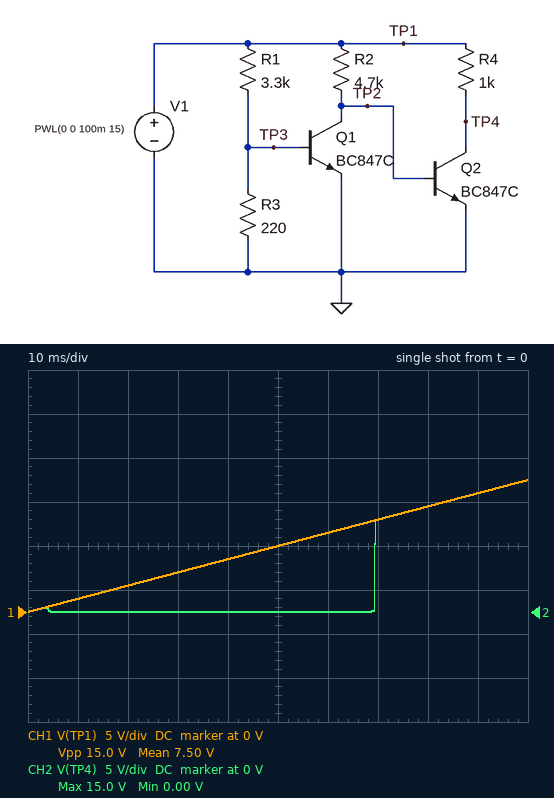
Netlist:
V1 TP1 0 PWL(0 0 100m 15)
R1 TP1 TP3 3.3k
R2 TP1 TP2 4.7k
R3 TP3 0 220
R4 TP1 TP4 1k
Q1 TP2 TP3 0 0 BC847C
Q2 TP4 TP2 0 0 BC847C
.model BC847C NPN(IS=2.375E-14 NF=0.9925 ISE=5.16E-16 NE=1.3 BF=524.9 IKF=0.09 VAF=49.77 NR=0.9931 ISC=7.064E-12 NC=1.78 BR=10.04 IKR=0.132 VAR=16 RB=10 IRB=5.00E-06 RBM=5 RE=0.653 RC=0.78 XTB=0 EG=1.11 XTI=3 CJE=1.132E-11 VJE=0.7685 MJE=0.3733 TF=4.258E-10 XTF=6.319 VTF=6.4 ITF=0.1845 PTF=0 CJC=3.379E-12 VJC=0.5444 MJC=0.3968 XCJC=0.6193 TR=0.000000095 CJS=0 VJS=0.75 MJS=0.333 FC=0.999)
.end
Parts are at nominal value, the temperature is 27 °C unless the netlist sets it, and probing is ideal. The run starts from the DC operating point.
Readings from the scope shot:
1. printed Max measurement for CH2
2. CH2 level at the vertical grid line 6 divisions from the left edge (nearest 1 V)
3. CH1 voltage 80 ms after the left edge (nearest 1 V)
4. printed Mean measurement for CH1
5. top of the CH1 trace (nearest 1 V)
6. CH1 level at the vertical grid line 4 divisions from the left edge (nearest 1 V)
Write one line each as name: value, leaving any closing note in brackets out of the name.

printed Max measurement for CH2: 15.0 V
CH2 level at the vertical grid line 6 divisions from the left edge: 0 V
CH1 voltage 80 ms after the left edge: 12 V
printed Mean measurement for CH1: 7.50 V
top of the CH1 trace: 15 V
CH1 level at the vertical grid line 4 divisions from the left edge: 6 V
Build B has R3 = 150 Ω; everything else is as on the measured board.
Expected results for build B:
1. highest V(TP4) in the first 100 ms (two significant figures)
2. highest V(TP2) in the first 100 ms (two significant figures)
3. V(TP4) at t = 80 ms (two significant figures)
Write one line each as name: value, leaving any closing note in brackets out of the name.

highest V(TP4) in the first 100 ms: 510 mV
highest V(TP2) in the first 100 ms: 750 mV
V(TP4) at t = 80 ms: 36 mV
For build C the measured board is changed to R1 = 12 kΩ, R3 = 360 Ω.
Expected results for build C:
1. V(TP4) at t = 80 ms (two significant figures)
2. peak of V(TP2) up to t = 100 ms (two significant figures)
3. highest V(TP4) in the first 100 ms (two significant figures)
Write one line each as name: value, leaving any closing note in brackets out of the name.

V(TP4) at t = 80 ms: 36 mV
peak of V(TP2) up to t = 100 ms: 760 mV
highest V(TP4) in the first 100 ms: 510 mV
